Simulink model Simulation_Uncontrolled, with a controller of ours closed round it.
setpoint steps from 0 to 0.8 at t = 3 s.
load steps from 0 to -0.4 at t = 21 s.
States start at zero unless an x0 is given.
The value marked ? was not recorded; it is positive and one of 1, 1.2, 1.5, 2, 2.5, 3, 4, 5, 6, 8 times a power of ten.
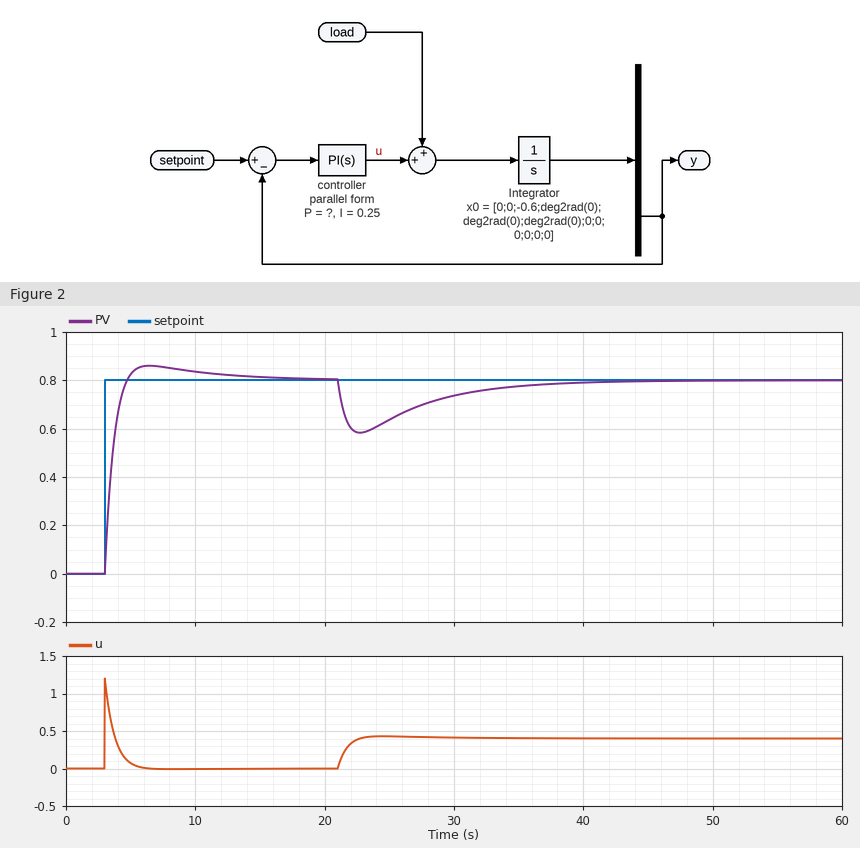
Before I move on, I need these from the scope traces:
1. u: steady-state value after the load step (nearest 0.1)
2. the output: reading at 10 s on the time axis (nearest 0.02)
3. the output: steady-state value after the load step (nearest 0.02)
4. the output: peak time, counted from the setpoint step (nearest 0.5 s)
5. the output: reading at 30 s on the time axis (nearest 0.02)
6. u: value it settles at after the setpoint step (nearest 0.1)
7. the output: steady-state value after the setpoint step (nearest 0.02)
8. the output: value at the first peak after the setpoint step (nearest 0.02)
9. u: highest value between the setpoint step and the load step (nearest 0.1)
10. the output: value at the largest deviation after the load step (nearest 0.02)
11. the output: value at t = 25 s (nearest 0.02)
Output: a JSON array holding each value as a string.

["0.4", "0.84", "0.80", "3.5 s", "0.74", "0.0", "0.80", "0.86", "1.2", "0.58", "0.64"]
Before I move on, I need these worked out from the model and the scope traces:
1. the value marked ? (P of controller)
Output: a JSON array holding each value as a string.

["1.5"]
